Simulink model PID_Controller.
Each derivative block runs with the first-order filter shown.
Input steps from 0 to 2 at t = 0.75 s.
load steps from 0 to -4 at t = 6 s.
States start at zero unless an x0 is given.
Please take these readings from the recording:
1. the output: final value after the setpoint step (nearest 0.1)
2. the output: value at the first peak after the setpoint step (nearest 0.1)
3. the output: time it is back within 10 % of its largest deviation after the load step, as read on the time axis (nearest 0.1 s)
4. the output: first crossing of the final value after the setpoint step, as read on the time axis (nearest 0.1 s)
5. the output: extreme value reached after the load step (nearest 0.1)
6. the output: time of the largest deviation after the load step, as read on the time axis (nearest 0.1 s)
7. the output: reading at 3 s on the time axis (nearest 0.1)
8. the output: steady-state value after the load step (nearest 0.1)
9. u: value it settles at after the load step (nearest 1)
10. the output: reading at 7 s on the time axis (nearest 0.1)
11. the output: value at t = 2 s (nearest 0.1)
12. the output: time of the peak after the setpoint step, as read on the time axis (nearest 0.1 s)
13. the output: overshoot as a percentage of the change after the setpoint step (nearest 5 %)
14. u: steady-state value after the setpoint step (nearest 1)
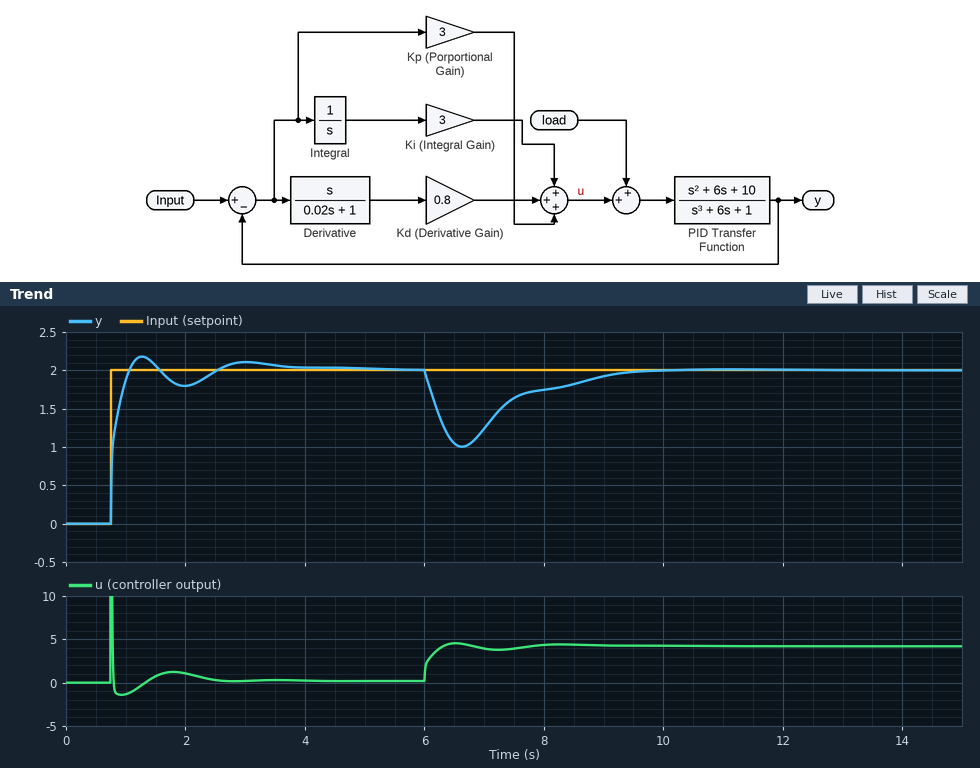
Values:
2.0
2.2
8.9 s
1.1 s
1.0
6.6 s
2.1
2.0
4
1.2
1.8
1.3 s
10 %
0
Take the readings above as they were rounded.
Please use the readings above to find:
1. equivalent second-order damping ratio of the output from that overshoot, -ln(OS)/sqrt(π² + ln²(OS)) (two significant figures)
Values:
0.59
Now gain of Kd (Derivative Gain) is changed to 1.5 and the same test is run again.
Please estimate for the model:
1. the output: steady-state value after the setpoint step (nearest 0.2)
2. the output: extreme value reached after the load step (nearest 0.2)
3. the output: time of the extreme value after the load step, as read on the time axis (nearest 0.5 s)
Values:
2.0
1.2
7.0 s
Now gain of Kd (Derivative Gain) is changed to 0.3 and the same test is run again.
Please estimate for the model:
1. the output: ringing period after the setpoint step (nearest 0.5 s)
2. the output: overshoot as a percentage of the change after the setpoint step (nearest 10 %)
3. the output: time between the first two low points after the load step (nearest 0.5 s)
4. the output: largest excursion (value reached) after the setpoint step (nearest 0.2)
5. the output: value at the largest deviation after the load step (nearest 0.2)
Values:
1.5 s
20 %
1.5 s
2.4
0.8
